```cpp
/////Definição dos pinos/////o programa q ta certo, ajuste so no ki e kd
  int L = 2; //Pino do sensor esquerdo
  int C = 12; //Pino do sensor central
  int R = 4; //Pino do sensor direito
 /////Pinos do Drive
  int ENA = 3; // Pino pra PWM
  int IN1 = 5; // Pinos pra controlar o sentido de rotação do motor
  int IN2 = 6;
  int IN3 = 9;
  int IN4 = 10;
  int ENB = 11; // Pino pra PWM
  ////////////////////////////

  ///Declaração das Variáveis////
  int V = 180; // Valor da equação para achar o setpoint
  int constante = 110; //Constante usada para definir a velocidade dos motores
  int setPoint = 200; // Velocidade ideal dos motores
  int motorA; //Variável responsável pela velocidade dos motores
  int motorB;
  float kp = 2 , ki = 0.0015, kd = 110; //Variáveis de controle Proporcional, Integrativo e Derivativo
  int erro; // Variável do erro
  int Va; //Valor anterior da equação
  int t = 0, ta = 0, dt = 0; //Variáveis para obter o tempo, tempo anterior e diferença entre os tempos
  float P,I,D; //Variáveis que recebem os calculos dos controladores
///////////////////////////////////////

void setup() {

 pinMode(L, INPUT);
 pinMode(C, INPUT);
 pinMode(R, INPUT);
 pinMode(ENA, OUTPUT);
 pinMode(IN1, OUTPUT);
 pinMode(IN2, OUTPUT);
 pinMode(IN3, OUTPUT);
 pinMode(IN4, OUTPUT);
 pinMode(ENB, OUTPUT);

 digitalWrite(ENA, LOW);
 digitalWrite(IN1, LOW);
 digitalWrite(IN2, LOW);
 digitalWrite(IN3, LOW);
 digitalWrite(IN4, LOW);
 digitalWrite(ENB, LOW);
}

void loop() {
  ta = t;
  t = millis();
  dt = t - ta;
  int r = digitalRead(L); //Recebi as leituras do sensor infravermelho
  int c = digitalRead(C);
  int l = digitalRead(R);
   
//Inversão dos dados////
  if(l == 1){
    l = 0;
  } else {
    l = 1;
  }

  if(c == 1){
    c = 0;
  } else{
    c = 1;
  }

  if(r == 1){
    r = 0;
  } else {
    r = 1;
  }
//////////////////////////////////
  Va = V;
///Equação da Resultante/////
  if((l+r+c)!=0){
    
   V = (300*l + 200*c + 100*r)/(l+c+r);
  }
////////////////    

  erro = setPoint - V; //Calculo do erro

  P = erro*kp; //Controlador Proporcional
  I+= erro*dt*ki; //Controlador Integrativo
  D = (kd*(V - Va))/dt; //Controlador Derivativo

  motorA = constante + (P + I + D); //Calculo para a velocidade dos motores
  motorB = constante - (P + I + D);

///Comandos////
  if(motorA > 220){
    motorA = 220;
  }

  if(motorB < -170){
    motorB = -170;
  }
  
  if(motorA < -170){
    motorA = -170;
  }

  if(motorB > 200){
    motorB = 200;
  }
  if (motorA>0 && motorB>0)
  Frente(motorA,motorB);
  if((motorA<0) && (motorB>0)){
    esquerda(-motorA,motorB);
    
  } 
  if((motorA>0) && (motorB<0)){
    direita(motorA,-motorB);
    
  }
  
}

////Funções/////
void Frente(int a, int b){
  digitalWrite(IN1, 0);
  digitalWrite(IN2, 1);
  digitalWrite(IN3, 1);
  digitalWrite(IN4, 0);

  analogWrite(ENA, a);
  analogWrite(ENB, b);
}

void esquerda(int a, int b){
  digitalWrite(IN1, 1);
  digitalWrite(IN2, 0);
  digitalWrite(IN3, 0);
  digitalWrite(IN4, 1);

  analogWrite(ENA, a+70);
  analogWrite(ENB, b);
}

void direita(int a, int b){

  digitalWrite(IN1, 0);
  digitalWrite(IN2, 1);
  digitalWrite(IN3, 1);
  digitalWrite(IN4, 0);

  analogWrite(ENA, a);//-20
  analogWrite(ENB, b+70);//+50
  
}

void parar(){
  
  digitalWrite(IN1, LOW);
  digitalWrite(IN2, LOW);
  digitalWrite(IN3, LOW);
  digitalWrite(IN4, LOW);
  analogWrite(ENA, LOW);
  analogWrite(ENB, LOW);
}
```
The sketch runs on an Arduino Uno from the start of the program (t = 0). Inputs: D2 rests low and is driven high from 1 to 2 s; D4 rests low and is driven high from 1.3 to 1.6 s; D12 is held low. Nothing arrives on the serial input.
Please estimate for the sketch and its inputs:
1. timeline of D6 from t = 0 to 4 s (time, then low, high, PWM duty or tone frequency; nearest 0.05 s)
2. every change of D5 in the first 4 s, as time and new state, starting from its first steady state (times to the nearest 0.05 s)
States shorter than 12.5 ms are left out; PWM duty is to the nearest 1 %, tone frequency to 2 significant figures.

0 s high; 1.15 s low; 1.3 s high; 1.6 s low; 2 s high
0 s low; 1.15 s high; 1.3 s low; 1.6 s high; 2 s low
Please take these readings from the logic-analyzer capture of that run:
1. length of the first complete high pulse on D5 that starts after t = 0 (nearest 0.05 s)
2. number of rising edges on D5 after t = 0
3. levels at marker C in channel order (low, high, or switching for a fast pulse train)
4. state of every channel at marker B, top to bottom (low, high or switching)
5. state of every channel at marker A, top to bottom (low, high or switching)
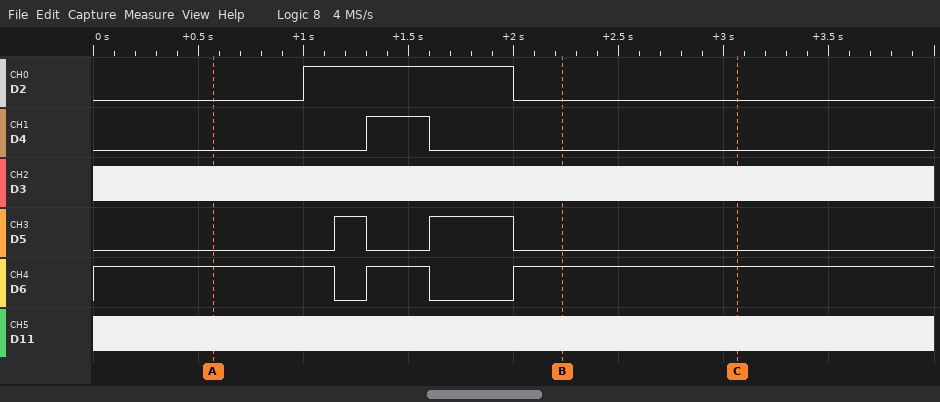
0.15 s
2
D2 low, D4 low, D3 switching, D5 low, D6 high, D11 switching
D2 low, D4 low, D3 switching, D5 low, D6 high, D11 switching
D2 low, D4 low, D3 switching, D5 low, D6 high, D11 switching
